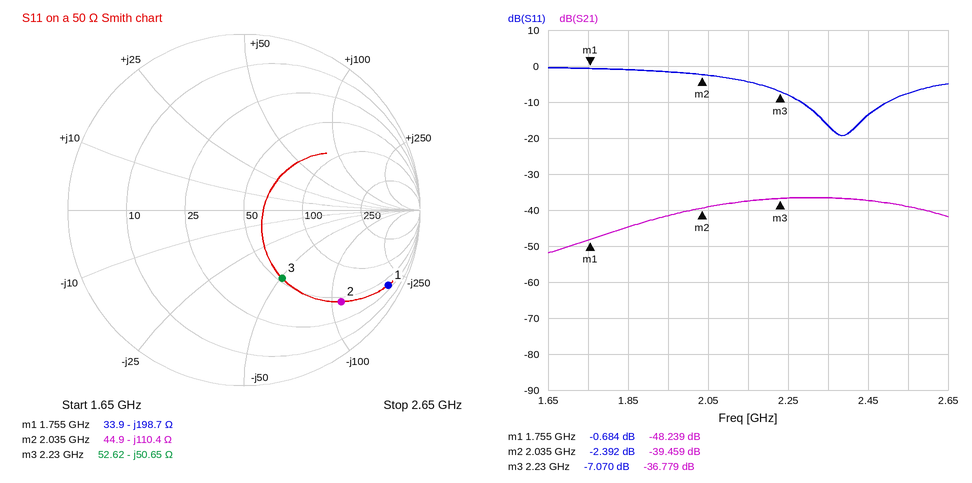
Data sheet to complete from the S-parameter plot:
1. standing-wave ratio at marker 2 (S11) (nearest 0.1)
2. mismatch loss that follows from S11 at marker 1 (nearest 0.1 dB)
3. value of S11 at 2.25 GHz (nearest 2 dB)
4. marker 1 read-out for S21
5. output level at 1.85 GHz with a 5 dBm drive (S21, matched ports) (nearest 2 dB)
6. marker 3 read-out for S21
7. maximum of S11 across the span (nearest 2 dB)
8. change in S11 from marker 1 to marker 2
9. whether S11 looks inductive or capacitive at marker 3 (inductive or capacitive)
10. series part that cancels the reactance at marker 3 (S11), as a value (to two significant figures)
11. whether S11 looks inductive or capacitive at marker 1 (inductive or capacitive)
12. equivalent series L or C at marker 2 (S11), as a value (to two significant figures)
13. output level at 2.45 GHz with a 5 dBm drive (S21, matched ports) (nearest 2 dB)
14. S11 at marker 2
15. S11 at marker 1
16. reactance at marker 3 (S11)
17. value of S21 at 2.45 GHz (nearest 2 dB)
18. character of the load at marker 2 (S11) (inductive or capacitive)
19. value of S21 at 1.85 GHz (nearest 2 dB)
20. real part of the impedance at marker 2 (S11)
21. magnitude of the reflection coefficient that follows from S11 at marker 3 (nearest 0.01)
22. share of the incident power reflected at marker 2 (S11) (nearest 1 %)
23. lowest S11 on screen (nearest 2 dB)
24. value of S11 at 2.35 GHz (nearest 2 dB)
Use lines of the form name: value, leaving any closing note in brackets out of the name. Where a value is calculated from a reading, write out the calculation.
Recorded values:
standing-wave ratio at marker 2 (S11): 7.3
mismatch loss that follows from S11 at marker 1: −10 log10(1 − 10^(-0.684/10)) ≈ 8.4 dB
value of S11 at 2.25 GHz: -8 dB
marker 1 read-out for S21: -48.239 dB
output level at 1.85 GHz with a 5 dBm drive (S21, matched ports): 5 dBm + (-44 dB) = -40 dBm
marker 3 read-out for S21: -36.779 dB
maximum of S11 across the span: 0 dB
change in S11 from marker 1 to marker 2: -2.392 − (-0.684) = -1.708 dB
whether S11 looks inductive or capacitive at marker 3: capacitive
series part that cancels the reactance at marker 3 (S11), as a value: L = 50.65 Ω/(2π × 2.23 GHz) ≈ 3.6 nH
whether S11 looks inductive or capacitive at marker 1: capacitive
equivalent series L or C at marker 2 (S11), as a value: C = 1/(2π × 2.035 GHz × 110.4 Ω) ≈ 708 fF, so 710 fF to two significant figures
output level at 2.45 GHz with a 5 dBm drive (S21, matched ports): 5 dBm + (-38 dB) = -32 dBm
S11 at marker 2: -2.392 dB
S11 at marker 1: -0.684 dB
reactance at marker 3: -50.65 Ω
value of S21 at 2.45 GHz: -38 dB
character of the load at marker 2 (S11): capacitive
value of S21 at 1.85 GHz: -44 dB
real part of the impedance at marker 2: 44.9 Ω
magnitude of the reflection coefficient that follows from S11 at marker 3: 10^(-7.07/20) ≈ 0.44
share of the incident power reflected at marker 2 (S11): 10^(-2.392/10) ≈ 58 %
lowest S11 on screen: -20 dB
value of S11 at 2.35 GHz: -16 dB
